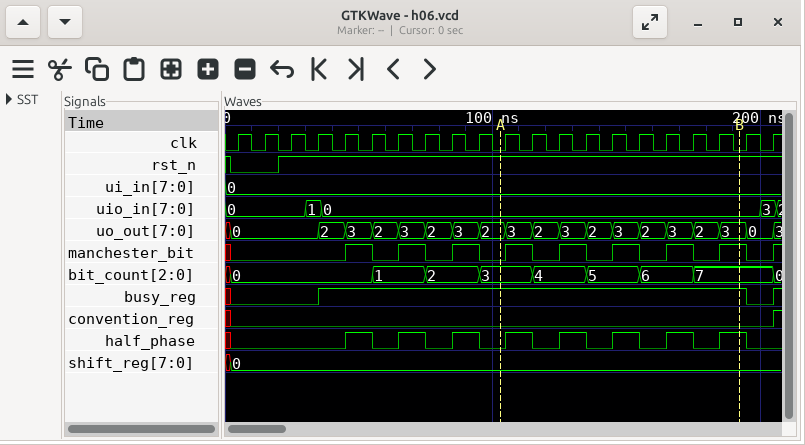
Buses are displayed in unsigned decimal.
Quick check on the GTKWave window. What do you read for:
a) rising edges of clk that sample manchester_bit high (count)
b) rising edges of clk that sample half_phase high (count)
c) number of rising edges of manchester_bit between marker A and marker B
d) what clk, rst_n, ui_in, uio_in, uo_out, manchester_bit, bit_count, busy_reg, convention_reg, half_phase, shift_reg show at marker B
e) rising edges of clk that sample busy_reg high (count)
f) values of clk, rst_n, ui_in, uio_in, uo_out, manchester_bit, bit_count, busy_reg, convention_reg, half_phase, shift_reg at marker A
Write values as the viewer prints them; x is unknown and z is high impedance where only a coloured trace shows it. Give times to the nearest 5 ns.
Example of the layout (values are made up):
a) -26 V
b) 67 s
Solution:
a) 8
b) 8
c) 5
d) clk=0, rst_n=1, ui_in=0, uio_in=0, uo_out=3, manchester_bit=1, bit_count=7, busy_reg=1, convention_reg=0, half_phase=1, shift_reg=0
e) 16
f) clk=0, rst_n=1, ui_in=0, uio_in=0, uo_out=2, manchester_bit=0, bit_count=3, busy_reg=1, convention_reg=0, half_phase=0, shift_reg=0
